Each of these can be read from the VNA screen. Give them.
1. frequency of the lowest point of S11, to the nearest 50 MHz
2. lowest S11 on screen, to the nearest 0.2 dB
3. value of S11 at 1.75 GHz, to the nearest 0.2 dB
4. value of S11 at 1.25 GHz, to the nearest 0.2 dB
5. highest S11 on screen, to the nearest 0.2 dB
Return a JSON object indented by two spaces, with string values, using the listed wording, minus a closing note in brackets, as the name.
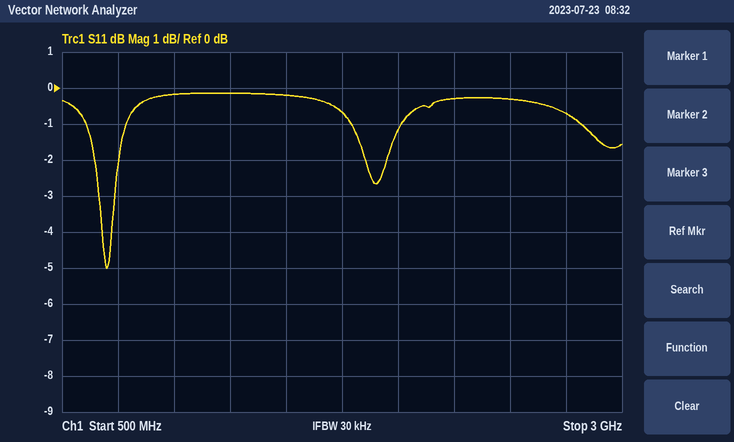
{
  "frequency of the lowest point of S11, to the nearest 50 MHz": "700 MHz",
  "lowest S11 on screen, to the nearest 0.2 dB": "-5.0 dB",
  "value of S11 at 1.75 GHz, to the nearest 0.2 dB": "-0.6 dB",
  "value of S11 at 1.25 GHz, to the nearest 0.2 dB": "-0.2 dB",
  "highest S11 on screen, to the nearest 0.2 dB": "-0.2 dB"
}
